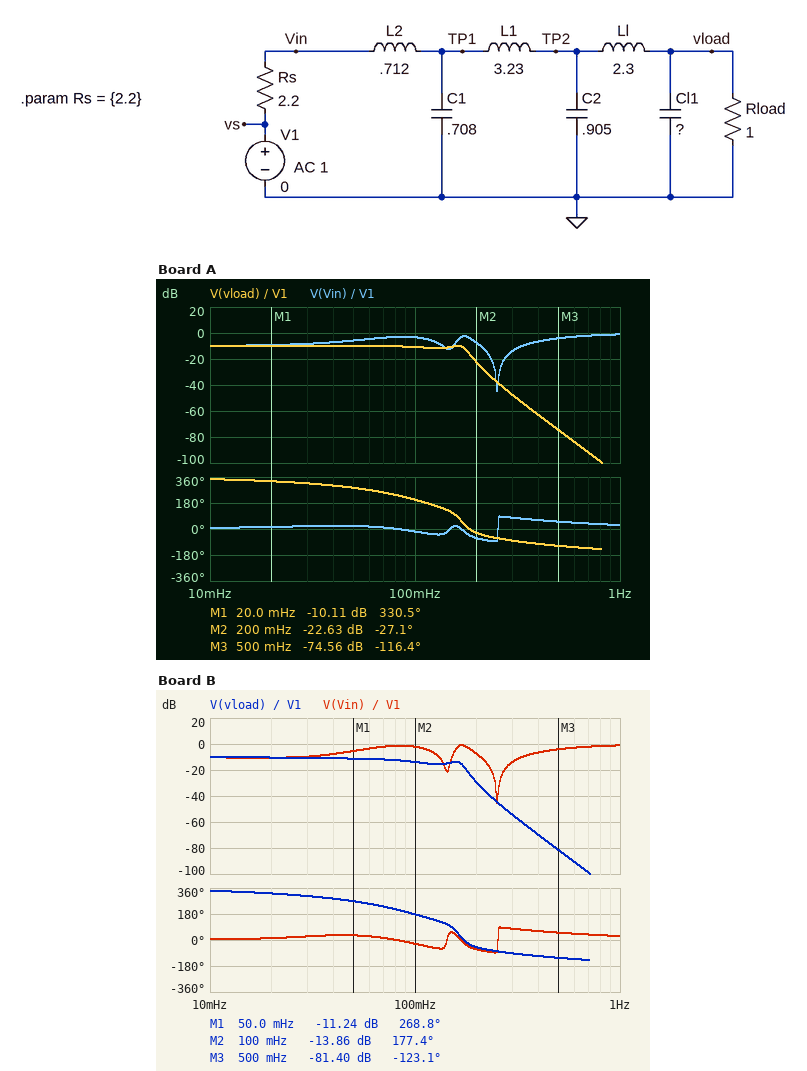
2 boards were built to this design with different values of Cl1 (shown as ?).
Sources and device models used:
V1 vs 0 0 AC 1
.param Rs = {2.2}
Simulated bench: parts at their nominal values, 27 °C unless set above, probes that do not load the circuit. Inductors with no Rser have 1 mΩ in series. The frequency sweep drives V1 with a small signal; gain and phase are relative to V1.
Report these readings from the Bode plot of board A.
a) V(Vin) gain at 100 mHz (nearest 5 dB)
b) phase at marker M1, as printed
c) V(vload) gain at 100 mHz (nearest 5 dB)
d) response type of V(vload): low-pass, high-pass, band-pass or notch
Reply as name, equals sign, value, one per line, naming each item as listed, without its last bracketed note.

V(Vin) gain at 100 mHz = -5 dB
phase at marker M1, as printed = 330.5 deg
V(vload) gain at 100 mHz = -10 dB
response type of V(vload): low-pass, high-pass, band-pass or notch = low-pass
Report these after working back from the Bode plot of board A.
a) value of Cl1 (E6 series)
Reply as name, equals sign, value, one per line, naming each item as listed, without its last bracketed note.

value of Cl1 = 1.5 F
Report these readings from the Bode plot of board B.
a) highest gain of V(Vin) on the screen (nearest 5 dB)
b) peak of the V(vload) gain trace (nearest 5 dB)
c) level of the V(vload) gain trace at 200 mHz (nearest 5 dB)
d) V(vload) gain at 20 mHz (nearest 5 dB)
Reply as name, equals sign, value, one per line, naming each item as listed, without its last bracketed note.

highest gain of V(Vin) on the screen = 0 dB
peak of the V(vload) gain trace = -10 dB
level of the V(vload) gain trace at 200 mHz = -30 dB
V(vload) gain at 20 mHz = -10 dB
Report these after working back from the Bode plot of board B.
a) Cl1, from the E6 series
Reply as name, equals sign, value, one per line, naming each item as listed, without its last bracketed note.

Cl1, from the E6 series = 3.3 F
